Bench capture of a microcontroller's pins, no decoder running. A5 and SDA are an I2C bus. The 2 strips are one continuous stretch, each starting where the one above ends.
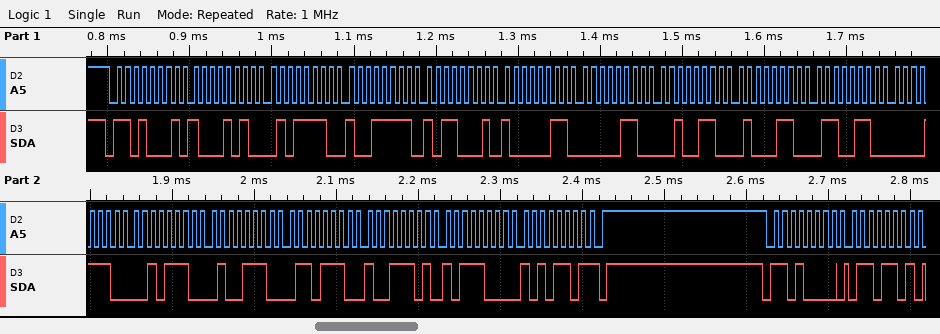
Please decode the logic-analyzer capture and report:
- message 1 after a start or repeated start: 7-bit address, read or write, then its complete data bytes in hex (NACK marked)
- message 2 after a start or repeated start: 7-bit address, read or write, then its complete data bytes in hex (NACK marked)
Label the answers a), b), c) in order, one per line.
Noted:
a) 0x68 read: 8A 5E 9F B1 83 06 26 46 66 0E 2E 4E 6E 9D B8 AD NACK
b) 0x68 write: 6D
